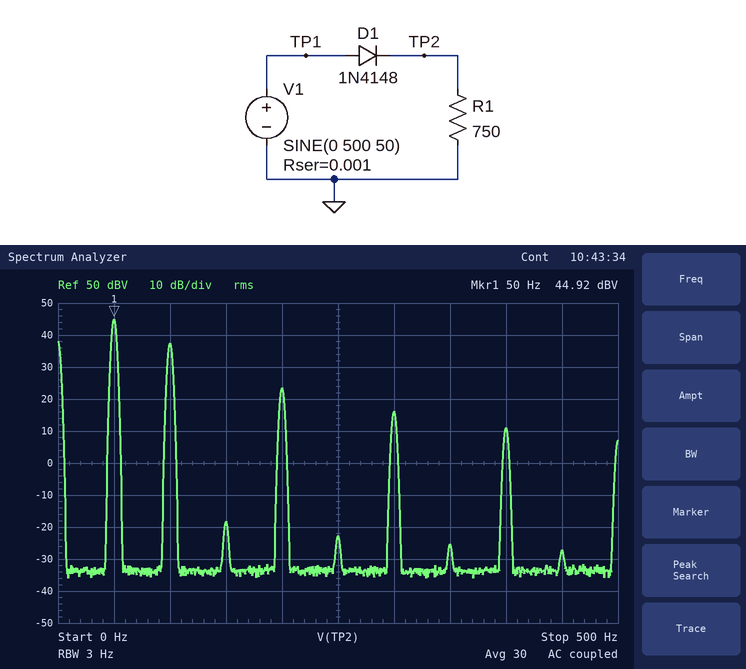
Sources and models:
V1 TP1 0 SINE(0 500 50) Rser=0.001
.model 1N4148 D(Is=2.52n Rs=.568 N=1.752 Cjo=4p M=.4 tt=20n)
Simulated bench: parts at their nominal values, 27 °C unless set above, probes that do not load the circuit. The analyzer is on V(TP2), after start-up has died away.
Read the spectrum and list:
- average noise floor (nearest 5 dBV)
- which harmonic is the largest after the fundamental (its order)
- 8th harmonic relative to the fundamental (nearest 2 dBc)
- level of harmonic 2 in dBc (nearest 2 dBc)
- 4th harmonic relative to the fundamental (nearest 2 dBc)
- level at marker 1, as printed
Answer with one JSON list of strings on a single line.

["-35 dBV", "2", "-34 dBc", "-8 dBc", "-22 dBc", "44.92 dBV"]
